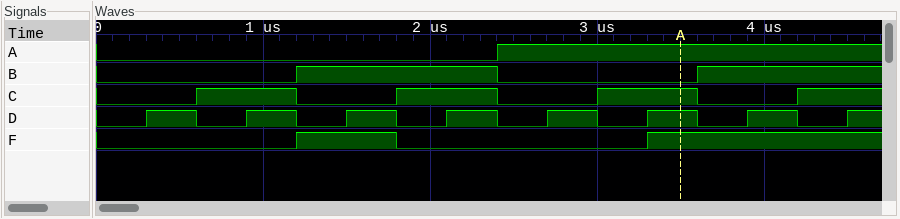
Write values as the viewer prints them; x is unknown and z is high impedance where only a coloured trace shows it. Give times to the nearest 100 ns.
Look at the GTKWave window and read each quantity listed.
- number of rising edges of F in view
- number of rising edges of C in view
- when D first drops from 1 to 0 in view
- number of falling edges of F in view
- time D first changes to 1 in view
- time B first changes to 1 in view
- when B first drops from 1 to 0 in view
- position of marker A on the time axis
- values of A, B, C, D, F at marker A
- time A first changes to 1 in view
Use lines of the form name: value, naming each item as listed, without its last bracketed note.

number of rising edges of F in view: 2
number of rising edges of C in view: 4
when D first drops from 1 to 0 in view: 600 ns
number of falling edges of F in view: 1
time D first changes to 1 in view: 300 ns
time B first changes to 1 in view: 1200 ns
when B first drops from 1 to 0 in view: 2400 ns
position of marker A on the time axis: 3500 ns
values of A, B, C, D, F at marker A: A=1, B=0, C=1, D=1, F=1
time A first changes to 1 in view: 2400 ns
